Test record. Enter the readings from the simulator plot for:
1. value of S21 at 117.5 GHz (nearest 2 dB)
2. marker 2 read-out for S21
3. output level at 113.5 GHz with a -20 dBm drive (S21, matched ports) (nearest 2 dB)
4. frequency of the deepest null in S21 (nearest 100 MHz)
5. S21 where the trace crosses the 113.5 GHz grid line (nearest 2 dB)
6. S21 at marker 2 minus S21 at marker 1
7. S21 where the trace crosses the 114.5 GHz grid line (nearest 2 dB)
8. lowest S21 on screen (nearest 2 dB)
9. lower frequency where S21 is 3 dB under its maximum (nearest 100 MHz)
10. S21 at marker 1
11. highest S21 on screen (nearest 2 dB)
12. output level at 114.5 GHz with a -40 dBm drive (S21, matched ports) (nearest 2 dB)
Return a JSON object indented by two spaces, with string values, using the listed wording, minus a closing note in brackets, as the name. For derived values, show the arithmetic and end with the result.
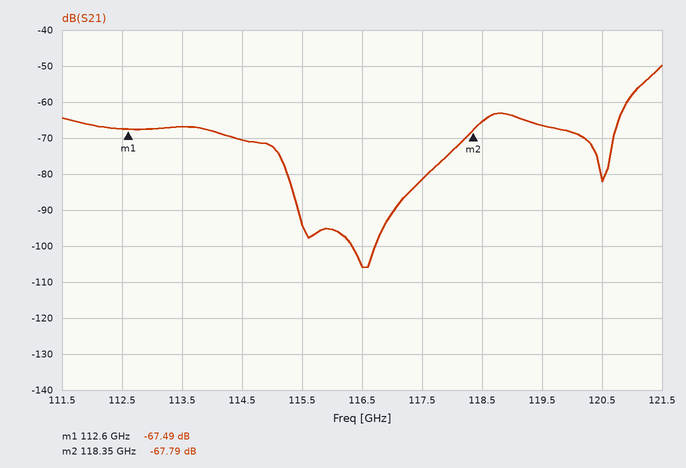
{
  "value of S21 at 117.5 GHz": "-82 dB",
  "marker 2 read-out for S21": "-67.79 dB",
  "output level at 113.5 GHz with a -20 dBm drive (S21, matched ports)": "-20 dBm + (-66 dB) = -86 dBm",
  "frequency of the deepest null in S21": "116.5 GHz",
  "S21 where the trace crosses the 113.5 GHz grid line": "-66 dB",
  "S21 at marker 2 minus S21 at marker 1": "-67.79 − (-67.49) = -0.30 dB",
  "S21 where the trace crosses the 114.5 GHz grid line": "-70 dB",
  "lowest S21 on screen": "-106 dB",
  "lower frequency where S21 is 3 dB under its maximum": "121.3 GHz",
  "S21 at marker 1": "-67.49 dB",
  "highest S21 on screen": "-50 dB",
  "output level at 114.5 GHz with a -40 dBm drive (S21, matched ports)": "-40 dBm + (-70 dB) = -110 dBm"
}
